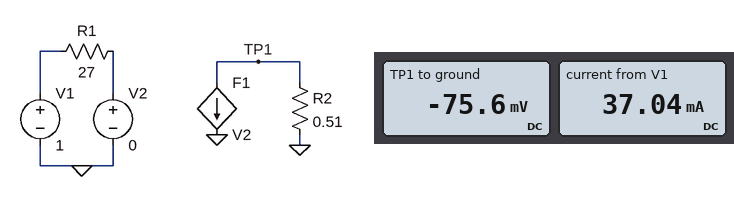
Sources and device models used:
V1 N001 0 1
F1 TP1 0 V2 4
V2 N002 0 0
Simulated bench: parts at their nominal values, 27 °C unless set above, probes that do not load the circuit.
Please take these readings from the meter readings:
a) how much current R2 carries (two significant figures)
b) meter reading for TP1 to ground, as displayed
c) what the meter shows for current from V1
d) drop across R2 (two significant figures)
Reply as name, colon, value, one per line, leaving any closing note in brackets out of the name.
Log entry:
how much current R2 carries: 150 mA
meter reading for TP1 to ground, as displayed: -75.6 mV
what the meter shows for current from V1: 37.04 mA
drop across R2: 76 mV
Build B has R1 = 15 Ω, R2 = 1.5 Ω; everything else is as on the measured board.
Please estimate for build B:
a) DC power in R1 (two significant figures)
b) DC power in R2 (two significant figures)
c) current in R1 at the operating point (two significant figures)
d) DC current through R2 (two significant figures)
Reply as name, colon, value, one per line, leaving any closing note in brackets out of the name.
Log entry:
DC power in R1: 67 mW
DC power in R2: 110 mW
current in R1 at the operating point: 67 mA
DC current through R2: 270 mA
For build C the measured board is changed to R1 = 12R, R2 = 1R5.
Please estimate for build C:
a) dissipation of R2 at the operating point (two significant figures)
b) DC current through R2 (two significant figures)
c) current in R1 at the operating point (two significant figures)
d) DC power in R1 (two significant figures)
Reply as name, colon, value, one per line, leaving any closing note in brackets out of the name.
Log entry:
dissipation of R2 at the operating point: 170 mW
DC current through R2: 330 mA
current in R1 at the operating point: 83 mA
DC power in R1: 83 mW
